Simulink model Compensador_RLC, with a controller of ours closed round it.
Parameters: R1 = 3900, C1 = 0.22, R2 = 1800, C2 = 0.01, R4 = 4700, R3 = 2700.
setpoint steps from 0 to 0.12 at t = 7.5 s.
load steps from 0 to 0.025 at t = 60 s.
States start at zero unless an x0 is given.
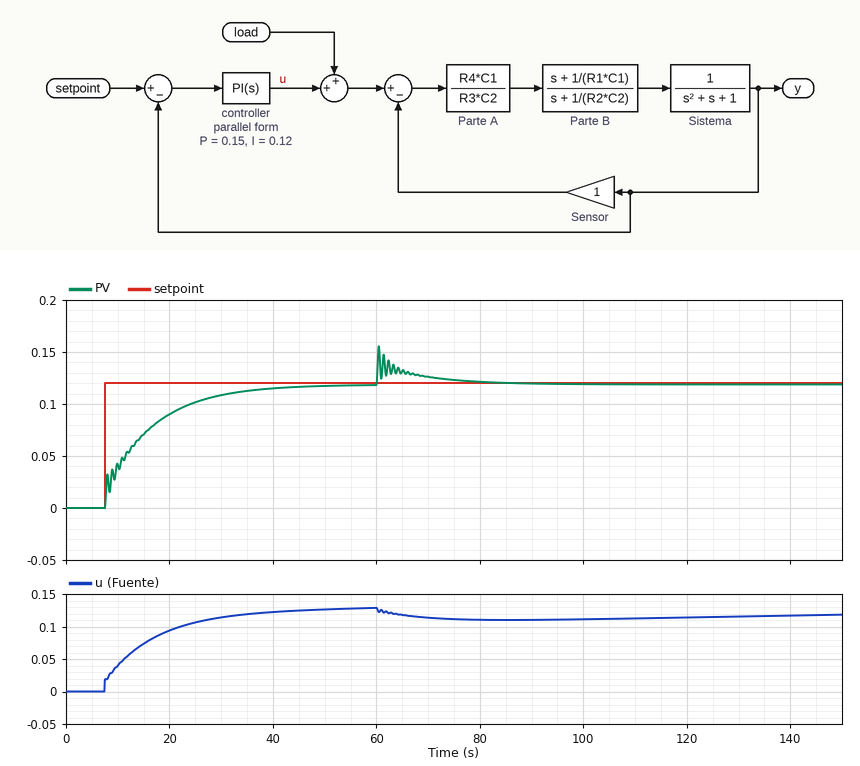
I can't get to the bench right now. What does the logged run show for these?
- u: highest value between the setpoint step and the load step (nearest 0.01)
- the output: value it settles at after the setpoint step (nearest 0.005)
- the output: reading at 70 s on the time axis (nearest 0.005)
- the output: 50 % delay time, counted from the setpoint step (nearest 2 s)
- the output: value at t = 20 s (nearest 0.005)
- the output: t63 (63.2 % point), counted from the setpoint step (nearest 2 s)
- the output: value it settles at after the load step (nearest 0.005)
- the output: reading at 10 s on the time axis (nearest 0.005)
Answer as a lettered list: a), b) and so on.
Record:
a) 0.13
b) 0.120
c) 0.125
d) 6 s
e) 0.090
f) 8 s
g) 0.120
h) 0.040
